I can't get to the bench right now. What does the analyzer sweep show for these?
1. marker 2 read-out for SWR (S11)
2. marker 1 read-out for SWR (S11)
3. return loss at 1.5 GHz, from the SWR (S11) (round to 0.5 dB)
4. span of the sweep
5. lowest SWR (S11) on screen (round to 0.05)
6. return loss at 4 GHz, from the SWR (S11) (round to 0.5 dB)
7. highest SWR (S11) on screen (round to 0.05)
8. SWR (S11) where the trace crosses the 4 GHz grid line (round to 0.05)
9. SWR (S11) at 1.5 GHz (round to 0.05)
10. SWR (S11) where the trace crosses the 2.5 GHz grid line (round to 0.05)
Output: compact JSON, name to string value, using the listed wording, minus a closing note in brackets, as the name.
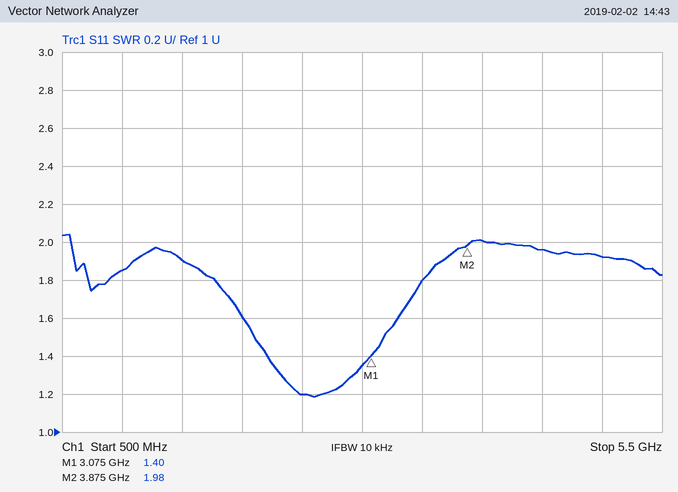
{"marker 2 read-out for SWR": "1.98", "marker 1 read-out for SWR": "1.40", "return loss at 1.5 GHz, from the SWR (S11)": "10.0 dB", "span of the sweep": "5 GHz", "lowest SWR (S11) on screen": "1.20", "return loss at 4 GHz, from the SWR (S11)": "9.5 dB", "highest SWR (S11) on screen": "2.05", "SWR (S11) where the trace crosses the 4 GHz grid line": "2.00", "SWR (S11) at 1.5 GHz": "1.90", "SWR (S11) where the trace crosses the 2.5 GHz grid line": "1.20"}
